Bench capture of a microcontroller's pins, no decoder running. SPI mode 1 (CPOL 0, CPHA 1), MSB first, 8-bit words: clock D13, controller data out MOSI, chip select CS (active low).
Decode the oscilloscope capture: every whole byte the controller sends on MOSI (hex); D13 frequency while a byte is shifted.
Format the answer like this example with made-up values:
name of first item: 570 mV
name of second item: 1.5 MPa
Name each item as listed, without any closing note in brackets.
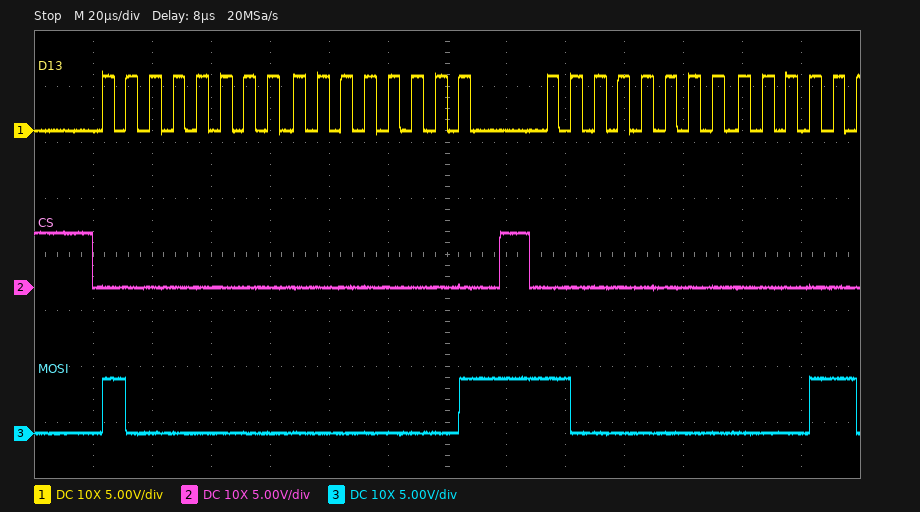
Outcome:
every whole byte the controller sends on MOSI: 80 01 80
D13 frequency while a byte is shifted: 125 kHz
